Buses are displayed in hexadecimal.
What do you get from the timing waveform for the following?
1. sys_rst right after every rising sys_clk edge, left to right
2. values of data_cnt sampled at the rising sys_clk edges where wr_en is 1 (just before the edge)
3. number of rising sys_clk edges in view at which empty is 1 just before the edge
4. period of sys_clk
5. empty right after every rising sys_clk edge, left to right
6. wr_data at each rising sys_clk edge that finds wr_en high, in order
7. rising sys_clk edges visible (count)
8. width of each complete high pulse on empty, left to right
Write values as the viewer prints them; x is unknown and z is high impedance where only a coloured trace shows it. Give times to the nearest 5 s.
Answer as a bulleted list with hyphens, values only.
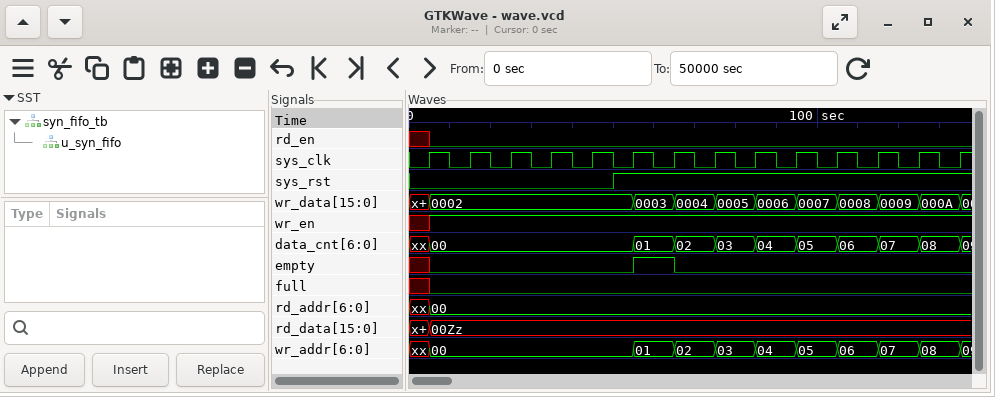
- 0 0 0 0 0 1 1 1 1 1 1 1 1 1
- 00, 00, 00, 00, 00, 01, 02, 03, 04, 05, 06, 07, 08
- 1
- 10 s
- 0 0 0 0 0 1 0 0 0 0 0 0 0 0
- 0002, 0002, 0002, 0002, 0002, 0003, 0004, 0005, 0006, 0007, 0008, 0009, 000A
- 14
- 10 s
